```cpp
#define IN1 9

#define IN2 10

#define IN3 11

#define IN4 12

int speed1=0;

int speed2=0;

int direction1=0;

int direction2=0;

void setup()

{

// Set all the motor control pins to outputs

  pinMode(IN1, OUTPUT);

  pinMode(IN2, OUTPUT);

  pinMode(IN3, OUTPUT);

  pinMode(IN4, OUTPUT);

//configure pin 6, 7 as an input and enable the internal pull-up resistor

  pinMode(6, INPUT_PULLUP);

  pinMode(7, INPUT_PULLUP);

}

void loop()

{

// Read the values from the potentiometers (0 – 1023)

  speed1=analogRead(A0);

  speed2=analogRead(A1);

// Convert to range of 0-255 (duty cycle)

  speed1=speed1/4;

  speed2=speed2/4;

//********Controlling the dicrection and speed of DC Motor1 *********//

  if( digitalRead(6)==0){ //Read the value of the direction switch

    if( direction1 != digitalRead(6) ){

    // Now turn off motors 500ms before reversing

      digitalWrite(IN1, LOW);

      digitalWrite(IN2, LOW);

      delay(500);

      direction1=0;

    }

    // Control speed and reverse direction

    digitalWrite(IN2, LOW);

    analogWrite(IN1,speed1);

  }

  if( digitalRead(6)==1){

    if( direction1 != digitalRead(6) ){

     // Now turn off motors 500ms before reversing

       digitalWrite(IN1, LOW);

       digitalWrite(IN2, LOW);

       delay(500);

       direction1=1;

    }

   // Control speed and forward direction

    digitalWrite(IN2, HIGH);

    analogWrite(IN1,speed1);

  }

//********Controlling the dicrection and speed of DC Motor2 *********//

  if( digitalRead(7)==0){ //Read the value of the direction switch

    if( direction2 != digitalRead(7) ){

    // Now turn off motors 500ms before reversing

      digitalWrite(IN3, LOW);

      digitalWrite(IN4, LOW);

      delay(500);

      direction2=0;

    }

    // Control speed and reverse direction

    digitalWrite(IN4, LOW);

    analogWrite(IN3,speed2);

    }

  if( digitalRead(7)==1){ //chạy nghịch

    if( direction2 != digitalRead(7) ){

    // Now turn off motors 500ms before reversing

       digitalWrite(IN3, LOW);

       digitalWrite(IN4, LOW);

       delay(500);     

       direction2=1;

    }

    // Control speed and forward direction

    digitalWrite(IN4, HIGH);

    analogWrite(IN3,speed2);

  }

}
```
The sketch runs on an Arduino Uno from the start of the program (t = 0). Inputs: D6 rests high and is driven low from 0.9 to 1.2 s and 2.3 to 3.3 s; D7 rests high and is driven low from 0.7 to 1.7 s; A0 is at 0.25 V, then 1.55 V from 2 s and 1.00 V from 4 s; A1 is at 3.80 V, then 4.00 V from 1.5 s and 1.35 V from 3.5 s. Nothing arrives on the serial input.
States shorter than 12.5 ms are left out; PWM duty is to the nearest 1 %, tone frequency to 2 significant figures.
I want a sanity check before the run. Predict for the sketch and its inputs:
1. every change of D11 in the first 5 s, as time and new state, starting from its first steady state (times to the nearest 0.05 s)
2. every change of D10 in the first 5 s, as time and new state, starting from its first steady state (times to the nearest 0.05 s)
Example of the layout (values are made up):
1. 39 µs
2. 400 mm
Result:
1. 0 s low; 1 s PWM 76 %; 2 s PWM 80 %; 3.8 s PWM 27 %
2. 0 s low; 0.5 s high; 1 s low; 2 s high; 2.3 s low; 3.8 s high
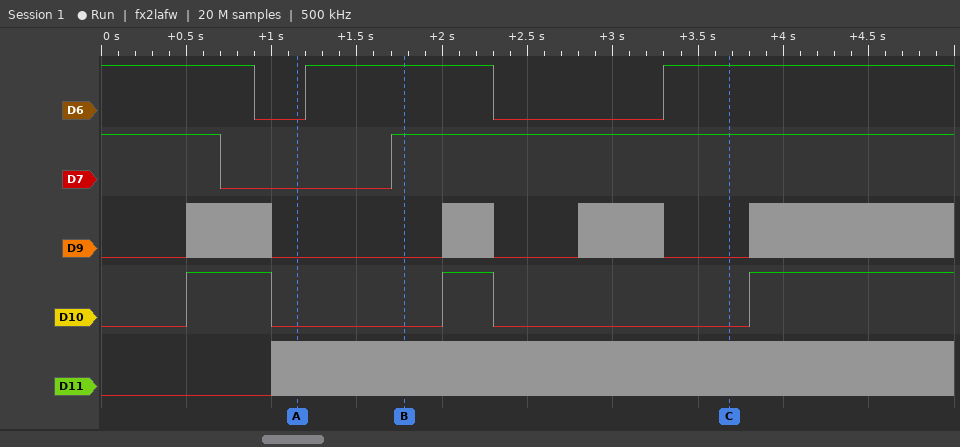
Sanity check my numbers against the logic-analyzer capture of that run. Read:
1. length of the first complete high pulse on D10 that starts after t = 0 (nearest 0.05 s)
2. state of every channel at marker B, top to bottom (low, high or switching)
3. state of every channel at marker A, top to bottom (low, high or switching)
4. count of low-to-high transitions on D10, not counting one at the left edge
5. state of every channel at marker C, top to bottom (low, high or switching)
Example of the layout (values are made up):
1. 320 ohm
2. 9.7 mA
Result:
1. 0.50 s
2. D6 high, D7 high, D9 low, D10 low, D11 switching
3. D6 low, D7 low, D9 low, D10 low, D11 switching
4. 3
5. D6 high, D7 high, D9 low, D10 low, D11 switching
